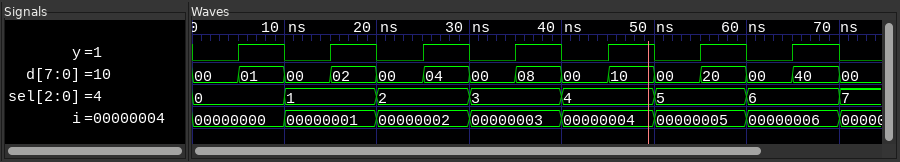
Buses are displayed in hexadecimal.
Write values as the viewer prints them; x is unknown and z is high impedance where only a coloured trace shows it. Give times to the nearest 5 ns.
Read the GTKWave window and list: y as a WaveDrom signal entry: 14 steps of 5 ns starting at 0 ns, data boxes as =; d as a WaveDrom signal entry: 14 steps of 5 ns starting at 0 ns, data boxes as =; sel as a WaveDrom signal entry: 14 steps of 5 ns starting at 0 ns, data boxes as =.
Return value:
{name: 'y', wave: '01010101010101'}
{name: 'd', wave: '==============', data: '00 01 00 02 00 04 00 08 00 10 00 20 00 40'}
{name: 'sel', wave: '=.=.=.=.=.=.=.', data: '0 1 2 3 4 5 6'}
